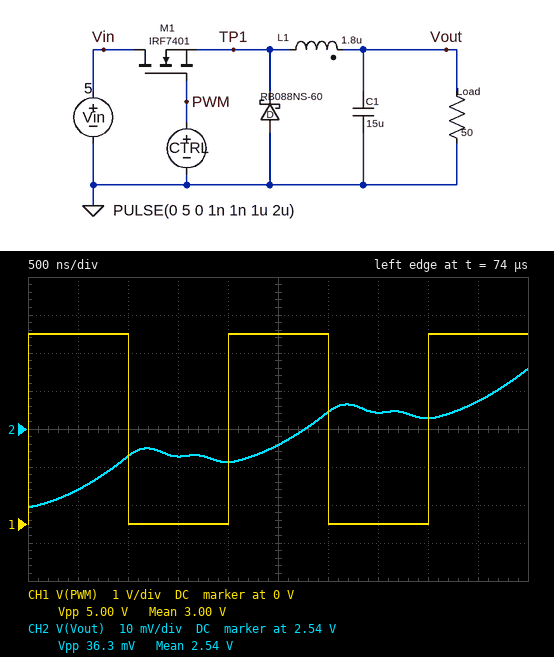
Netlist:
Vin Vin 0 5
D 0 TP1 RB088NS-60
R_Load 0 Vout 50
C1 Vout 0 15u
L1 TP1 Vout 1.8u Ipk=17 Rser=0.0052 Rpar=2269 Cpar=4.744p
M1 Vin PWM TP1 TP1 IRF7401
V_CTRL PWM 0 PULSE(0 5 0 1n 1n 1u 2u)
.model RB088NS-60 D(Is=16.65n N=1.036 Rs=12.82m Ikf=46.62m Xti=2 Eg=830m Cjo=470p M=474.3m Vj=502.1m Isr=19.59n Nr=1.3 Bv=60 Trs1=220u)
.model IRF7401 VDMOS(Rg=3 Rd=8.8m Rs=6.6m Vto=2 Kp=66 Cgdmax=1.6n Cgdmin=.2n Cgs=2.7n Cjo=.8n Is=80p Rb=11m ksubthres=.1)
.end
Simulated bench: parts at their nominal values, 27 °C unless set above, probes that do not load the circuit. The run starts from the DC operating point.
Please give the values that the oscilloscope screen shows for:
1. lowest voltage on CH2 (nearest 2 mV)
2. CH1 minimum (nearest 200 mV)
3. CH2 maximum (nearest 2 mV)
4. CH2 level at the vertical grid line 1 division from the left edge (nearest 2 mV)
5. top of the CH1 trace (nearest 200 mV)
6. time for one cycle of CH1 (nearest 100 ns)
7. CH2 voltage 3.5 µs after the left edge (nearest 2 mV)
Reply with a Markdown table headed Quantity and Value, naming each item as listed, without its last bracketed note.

| Quantity | Value |
|---|---|
| lowest voltage on CH2 | 2.520 V |
| CH1 minimum | 0 V |
| CH2 maximum | 2.556 V |
| CH2 level at the vertical grid line 1 division from the left edge | 2.524 V |
| top of the CH1 trace | 5.0 V |
| time for one cycle of CH1 | 2.0 µs |
| CH2 voltage 3.5 µs after the left edge | 2.544 V |
